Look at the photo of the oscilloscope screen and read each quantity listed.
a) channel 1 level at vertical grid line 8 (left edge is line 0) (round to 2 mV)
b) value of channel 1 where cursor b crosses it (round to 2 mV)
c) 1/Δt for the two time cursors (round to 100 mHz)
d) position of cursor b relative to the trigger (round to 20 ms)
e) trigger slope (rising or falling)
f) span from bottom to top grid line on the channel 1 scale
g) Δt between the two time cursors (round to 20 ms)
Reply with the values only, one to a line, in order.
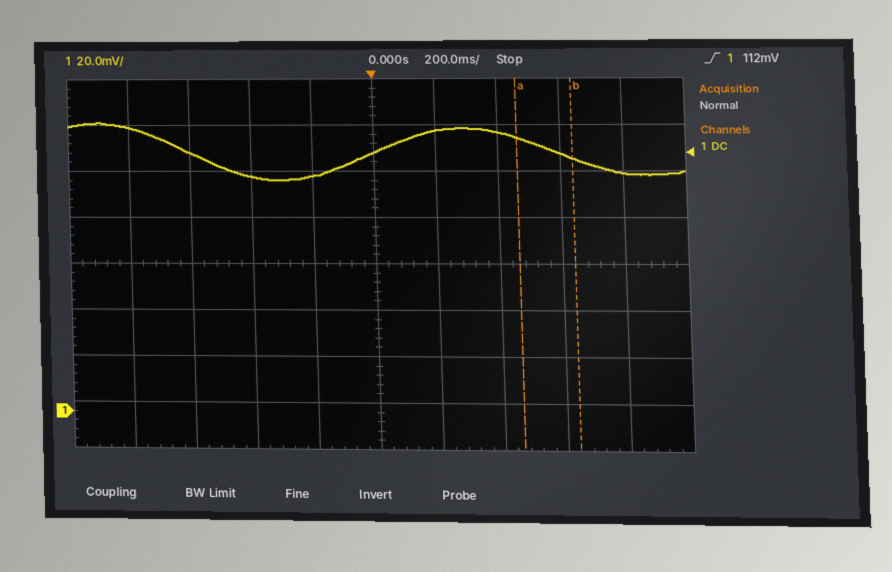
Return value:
112 mV
110 mV
5.6 Hz
+640 ms
rising
160 mV
180 ms
